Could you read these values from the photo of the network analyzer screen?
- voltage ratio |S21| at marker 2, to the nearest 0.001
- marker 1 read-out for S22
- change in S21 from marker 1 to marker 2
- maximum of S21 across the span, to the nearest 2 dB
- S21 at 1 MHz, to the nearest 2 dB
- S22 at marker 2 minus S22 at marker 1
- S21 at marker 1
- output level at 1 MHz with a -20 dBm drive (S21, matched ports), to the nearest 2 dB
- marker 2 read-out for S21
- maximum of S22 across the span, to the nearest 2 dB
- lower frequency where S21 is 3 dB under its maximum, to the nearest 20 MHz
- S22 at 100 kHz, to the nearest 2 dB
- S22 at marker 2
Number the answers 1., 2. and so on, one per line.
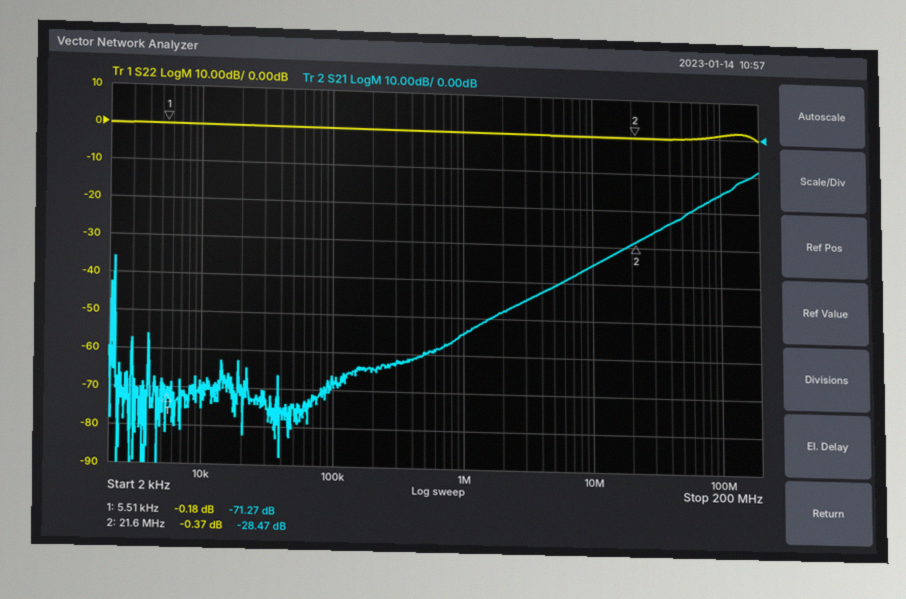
1. 0.038
2. -0.18 dB
3. 42.80 dB
4. -8 dB
5. -54 dB
6. -0.19 dB
7. -71.27 dB
8. -74 dBm
9. -28.47 dB
10. 2 dB
11. 140 MHz
12. 0 dB
13. -0.37 dB
